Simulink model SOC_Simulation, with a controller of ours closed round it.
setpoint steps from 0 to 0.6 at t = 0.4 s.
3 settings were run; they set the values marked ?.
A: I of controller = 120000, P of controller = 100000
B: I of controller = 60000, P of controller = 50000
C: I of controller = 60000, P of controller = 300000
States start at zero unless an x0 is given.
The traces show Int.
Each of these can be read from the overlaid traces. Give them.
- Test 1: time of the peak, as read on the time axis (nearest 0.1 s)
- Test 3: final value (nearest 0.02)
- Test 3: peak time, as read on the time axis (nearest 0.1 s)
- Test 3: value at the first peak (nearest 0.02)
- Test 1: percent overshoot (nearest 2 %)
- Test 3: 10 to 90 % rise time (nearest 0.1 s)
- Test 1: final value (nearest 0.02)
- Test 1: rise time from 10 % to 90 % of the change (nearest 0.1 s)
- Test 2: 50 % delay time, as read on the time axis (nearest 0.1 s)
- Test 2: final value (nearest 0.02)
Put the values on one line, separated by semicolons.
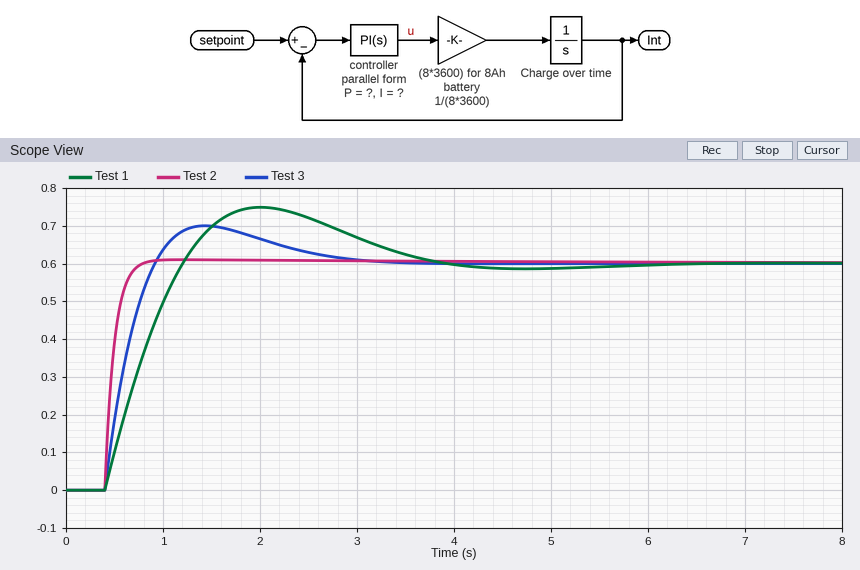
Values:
2.0 s; 0.60; 1.4 s; 0.70; 24 %; 0.4 s; 0.60; 0.6 s; 0.5 s; 0.60
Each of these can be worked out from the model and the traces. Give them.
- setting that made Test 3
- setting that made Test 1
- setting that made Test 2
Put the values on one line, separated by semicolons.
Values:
A; B; C
